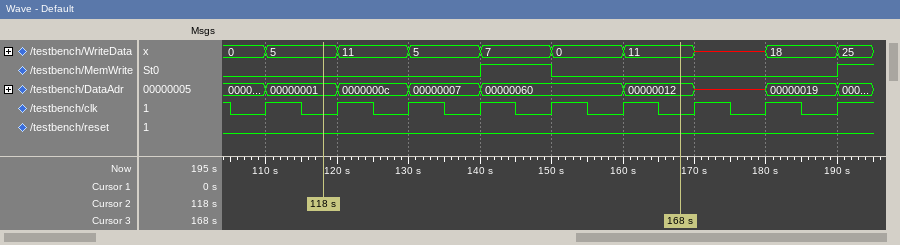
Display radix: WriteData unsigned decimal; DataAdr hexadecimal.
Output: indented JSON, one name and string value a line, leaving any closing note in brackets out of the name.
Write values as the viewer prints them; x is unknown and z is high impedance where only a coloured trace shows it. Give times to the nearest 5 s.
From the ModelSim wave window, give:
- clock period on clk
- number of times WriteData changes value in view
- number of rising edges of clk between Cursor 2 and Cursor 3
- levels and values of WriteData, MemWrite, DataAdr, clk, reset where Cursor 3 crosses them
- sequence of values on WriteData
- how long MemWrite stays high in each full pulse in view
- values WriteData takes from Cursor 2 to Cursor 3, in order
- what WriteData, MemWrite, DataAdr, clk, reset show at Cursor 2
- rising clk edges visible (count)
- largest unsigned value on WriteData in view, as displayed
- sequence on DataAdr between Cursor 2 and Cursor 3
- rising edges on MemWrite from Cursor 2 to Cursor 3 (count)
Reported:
{
  "clock period on clk": "10 s",
  "number of times WriteData changes value in view": "9",
  "number of rising edges of clk between Cursor 2 and Cursor 3": "5",
  "levels and values of WriteData, MemWrite, DataAdr, clk, reset where Cursor 3 crosses them": "WriteData=11, MemWrite=0, DataAdr=00000012, clk=0, reset=0",
  "sequence of values on WriteData": "0, 5, 11, 5, 7, 0, 11, x, 18, 25",
  "how long MemWrite stays high in each full pulse in view": "10 s",
  "values WriteData takes from Cursor 2 to Cursor 3, in order": "5, 11, 5, 7, 0, 11",
  "what WriteData, MemWrite, DataAdr, clk, reset show at Cursor 2": "WriteData=5, MemWrite=0, DataAdr=00000001, clk=0, reset=0",
  "rising clk edges visible": "9",
  "largest unsigned value on WriteData in view, as displayed": "25",
  "sequence on DataAdr between Cursor 2 and Cursor 3": "00000001, 0000000c, 00000007, 00000060, 00000012",
  "rising edges on MemWrite from Cursor 2 to Cursor 3": "1"
}
